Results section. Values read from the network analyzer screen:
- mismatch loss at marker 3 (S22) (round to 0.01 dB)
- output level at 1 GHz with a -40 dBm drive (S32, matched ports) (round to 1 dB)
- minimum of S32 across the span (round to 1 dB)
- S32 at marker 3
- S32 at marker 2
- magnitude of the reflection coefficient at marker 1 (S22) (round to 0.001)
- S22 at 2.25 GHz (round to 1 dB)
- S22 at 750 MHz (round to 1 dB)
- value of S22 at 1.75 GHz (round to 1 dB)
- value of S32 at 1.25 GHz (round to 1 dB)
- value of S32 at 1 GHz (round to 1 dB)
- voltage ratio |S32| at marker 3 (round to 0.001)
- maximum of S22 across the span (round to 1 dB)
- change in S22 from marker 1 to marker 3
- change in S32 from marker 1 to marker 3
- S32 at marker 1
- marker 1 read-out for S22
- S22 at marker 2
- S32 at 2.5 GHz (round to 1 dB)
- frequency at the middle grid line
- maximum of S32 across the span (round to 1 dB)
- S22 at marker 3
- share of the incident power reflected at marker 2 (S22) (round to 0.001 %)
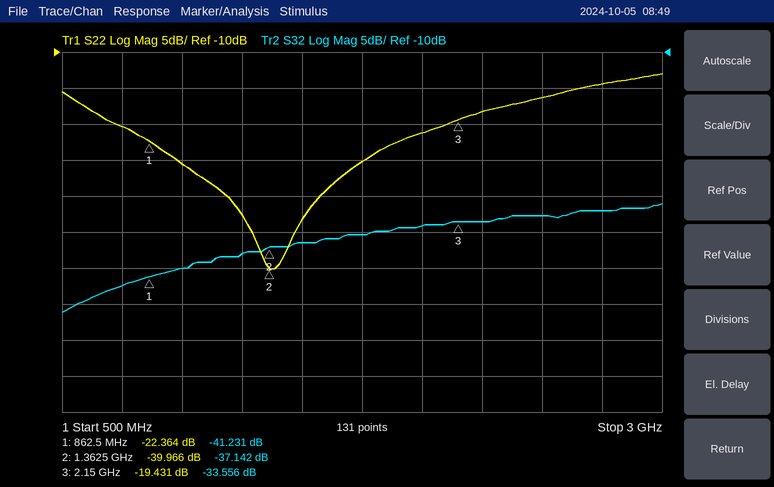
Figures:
0.05 dB
-80 dBm
-46 dB
-33.556 dB
-37.142 dB
0.076
-18 dB
-20 dB
-25 dB
-38 dB
-40 dB
0.021
-13 dB
2.933 dB
7.675 dB
-41.231 dB
-22.364 dB
-39.966 dB
-33 dB
1.75 GHz
-31 dB
-19.431 dB
0.010 %
